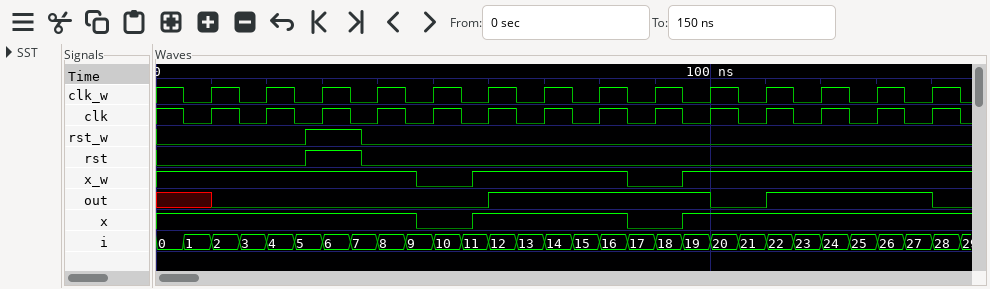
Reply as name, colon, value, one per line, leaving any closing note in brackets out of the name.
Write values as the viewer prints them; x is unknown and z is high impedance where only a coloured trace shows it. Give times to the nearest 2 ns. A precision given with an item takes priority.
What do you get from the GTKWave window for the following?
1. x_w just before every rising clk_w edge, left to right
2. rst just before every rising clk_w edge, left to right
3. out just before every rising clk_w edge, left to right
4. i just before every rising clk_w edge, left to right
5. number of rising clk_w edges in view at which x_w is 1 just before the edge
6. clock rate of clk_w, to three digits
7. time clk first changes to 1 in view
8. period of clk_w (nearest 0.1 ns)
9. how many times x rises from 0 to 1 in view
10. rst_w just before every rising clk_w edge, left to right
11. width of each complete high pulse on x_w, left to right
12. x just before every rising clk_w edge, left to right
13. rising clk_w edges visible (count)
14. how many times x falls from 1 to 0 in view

x_w just before every rising clk_w edge, left to right: 1 1 1 1 0 1 1 1 0 1 1 1 1 1
rst just before every rising clk_w edge, left to right: 0 0 1 0 0 0 0 0 0 0 0 0 0 0
out just before every rising clk_w edge, left to right: x 0 0 0 0 0 1 1 1 1 0 1 1 1
i just before every rising clk_w edge, left to right: 1, 3, 5, 7, 9, 11, 13, 15, 17, 19, 21, 23, 25, 27
number of rising clk_w edges in view at which x_w is 1 just before the edge: 12
clock rate of clk_w, to three digits: 100 MHz
time clk first changes to 1 in view: 10 ns
period of clk_w: 10 ns
how many times x rises from 0 to 1 in view: 2
rst_w just before every rising clk_w edge, left to right: 0 0 1 0 0 0 0 0 0 0 0 0 0 0
width of each complete high pulse on x_w, left to right: 28 ns
x just before every rising clk_w edge, left to right: 1 1 1 1 0 1 1 1 0 1 1 1 1 1
rising clk_w edges visible: 14
how many times x falls from 1 to 0 in view: 2
